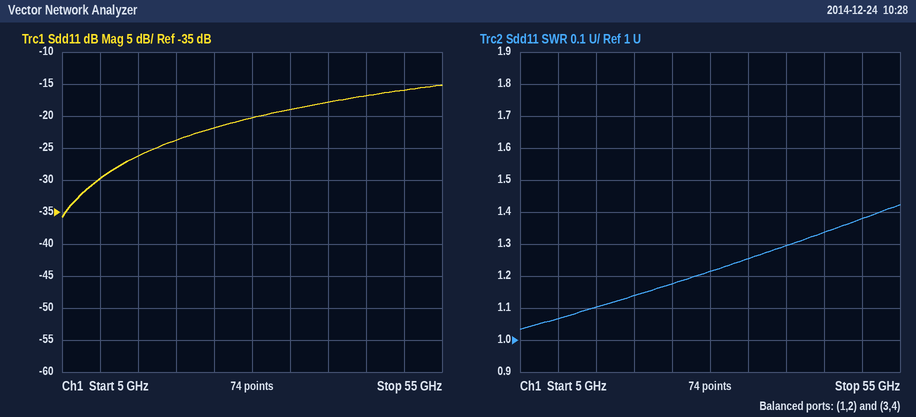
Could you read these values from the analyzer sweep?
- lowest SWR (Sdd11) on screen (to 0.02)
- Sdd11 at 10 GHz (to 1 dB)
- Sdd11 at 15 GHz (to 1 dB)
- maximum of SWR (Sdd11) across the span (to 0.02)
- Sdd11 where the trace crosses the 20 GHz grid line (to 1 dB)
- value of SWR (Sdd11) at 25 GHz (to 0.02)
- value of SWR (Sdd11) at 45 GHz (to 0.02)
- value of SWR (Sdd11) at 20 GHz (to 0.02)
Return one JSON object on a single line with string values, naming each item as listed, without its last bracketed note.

{"lowest SWR (Sdd11) on screen": "1.04", "Sdd11 at 10 GHz": "-30 dB", "Sdd11 at 15 GHz": "-26 dB", "maximum of SWR (Sdd11) across the span": "1.42", "Sdd11 where the trace crosses the 20 GHz grid line": "-24 dB", "value of SWR (Sdd11) at 25 GHz": "1.18", "value of SWR (Sdd11) at 45 GHz": "1.34", "value of SWR (Sdd11) at 20 GHz": "1.14"}
